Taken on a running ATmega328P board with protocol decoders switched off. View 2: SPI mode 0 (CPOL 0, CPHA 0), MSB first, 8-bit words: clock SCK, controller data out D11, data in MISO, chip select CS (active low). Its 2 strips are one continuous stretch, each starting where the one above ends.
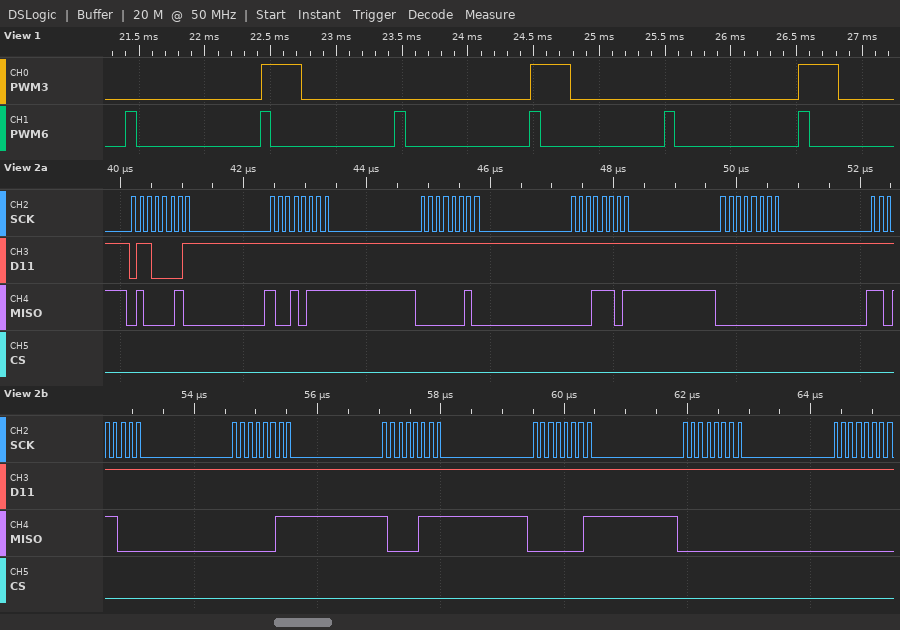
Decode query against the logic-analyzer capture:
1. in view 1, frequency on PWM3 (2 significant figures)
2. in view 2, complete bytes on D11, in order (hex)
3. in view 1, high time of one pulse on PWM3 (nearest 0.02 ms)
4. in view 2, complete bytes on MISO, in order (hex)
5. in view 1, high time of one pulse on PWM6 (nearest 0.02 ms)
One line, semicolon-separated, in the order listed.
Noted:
490 Hz; 61 FF FF FF FF FF FF FF FF FF FF; 0.30 ms; 42 97 02 1D 00 D8 03 87 01 00 00; 0.08 ms
